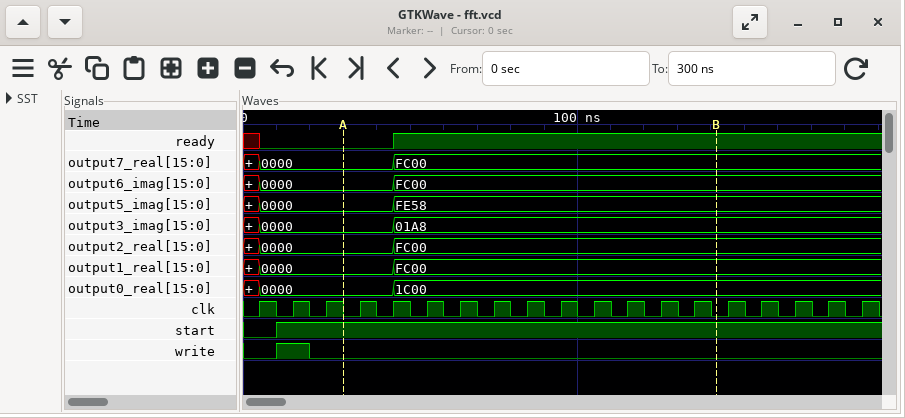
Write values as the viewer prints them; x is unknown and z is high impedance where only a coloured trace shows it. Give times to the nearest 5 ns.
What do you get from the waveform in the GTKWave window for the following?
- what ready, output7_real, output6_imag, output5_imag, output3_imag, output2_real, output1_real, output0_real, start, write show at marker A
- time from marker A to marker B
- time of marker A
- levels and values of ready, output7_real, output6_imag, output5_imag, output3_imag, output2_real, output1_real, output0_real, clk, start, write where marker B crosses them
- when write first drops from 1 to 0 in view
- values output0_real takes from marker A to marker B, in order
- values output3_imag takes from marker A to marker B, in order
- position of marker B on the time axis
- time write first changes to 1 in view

ready=0, output7_real=0000, output6_imag=0000, output5_imag=0000, output3_imag=0000, output2_real=0000, output1_real=0000, output0_real=0000, start=1, write=0
110 ns
30 ns
ready=1, output7_real=FC00, output6_imag=FC00, output5_imag=FE58, output3_imag=01A8, output2_real=FC00, output1_real=FC00, output0_real=1C00, clk=0, start=1, write=0
20 ns
0000, 1C00
0000, 01A8
140 ns
10 ns
